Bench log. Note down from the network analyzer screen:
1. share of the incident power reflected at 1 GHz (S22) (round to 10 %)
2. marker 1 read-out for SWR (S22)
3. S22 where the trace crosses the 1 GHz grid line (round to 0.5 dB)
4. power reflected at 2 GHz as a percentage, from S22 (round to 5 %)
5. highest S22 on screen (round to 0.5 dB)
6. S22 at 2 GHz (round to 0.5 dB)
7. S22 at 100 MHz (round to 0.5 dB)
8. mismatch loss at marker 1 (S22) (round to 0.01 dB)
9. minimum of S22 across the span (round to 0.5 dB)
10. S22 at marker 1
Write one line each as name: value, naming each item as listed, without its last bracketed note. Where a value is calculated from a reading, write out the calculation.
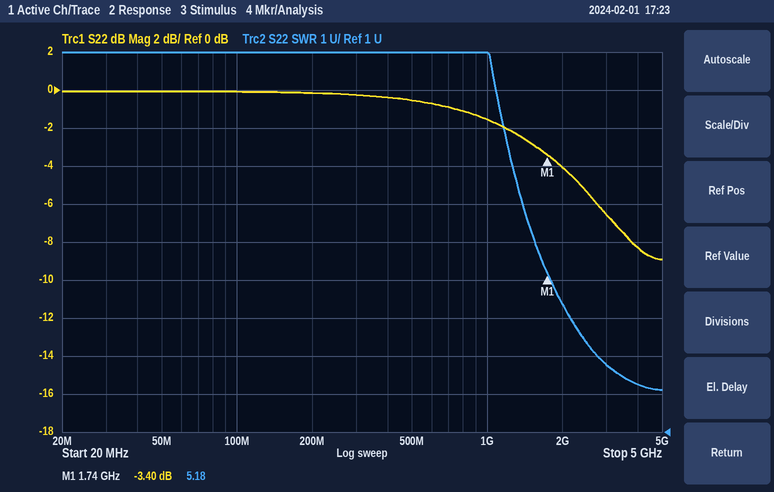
share of the incident power reflected at 1 GHz (S22): 10^(-1.5/10) ≈ 70.8 %, so 70 % to the nearest 10 %
marker 1 read-out for SWR: 5.18
S22 where the trace crosses the 1 GHz grid line: -1.5 dB
power reflected at 2 GHz as a percentage, from S22: 10^(-4/10) ≈ 40 %
highest S22 on screen: 0.0 dB
S22 at 2 GHz: -4.0 dB
S22 at 100 MHz: 0.0 dB
mismatch loss at marker 1 (S22): −10 log10(1 − 10^(-3.4/10)) ≈ 2.65 dB
minimum of S22 across the span: -9.0 dB
S22 at marker 1: -3.40 dB
